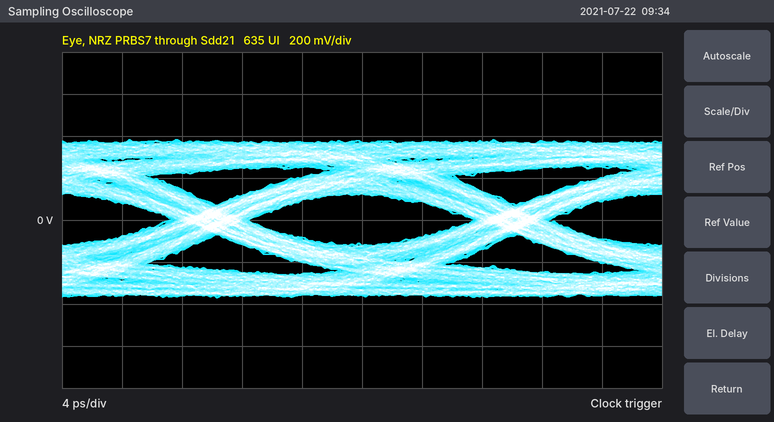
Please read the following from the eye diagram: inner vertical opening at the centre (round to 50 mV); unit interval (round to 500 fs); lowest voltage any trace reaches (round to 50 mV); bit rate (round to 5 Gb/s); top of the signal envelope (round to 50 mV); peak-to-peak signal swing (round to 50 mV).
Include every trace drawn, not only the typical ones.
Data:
250 mV
20.0 ps
-350 mV
50 Gb/s
400 mV
750 mV
